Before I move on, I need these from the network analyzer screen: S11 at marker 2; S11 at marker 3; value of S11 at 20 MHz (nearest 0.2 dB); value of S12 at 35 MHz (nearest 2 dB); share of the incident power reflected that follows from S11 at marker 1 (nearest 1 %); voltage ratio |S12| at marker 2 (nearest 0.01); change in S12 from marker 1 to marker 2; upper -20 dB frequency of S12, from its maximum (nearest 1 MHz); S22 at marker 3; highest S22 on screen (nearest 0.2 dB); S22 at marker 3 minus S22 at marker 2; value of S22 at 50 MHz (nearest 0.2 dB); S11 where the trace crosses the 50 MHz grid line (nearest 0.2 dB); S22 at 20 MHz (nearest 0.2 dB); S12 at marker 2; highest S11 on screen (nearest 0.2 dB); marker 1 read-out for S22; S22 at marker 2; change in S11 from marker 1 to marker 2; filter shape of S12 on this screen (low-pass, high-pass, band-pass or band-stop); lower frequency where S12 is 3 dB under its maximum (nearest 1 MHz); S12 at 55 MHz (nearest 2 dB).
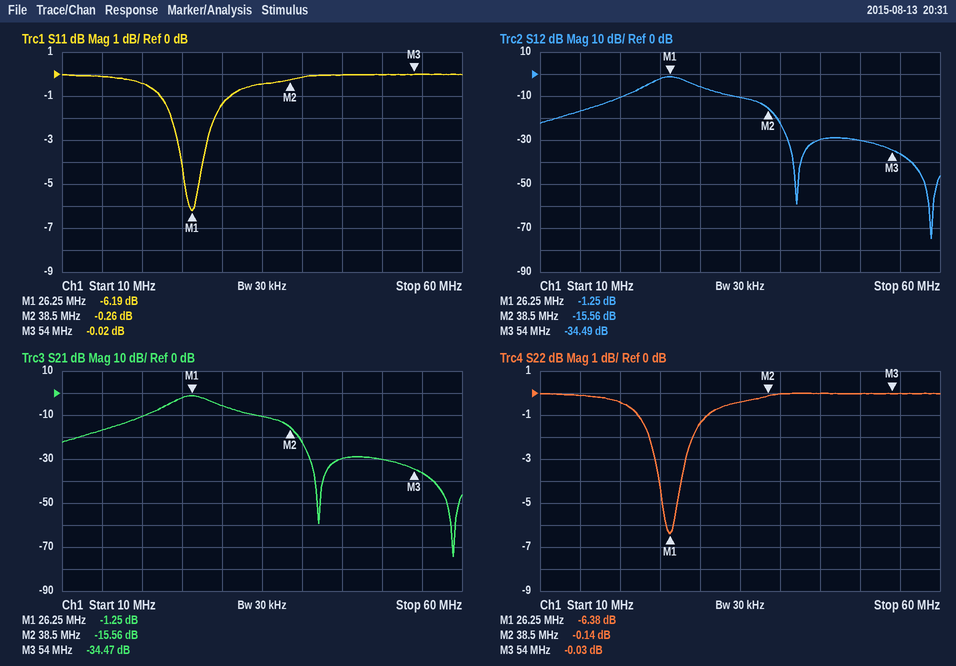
-0.26 dB
-0.02 dB
-0.4 dB
-10 dB
24 %
0.17
-14.31 dB
40 MHz
-0.03 dB
0.0 dB
0.11 dB
0.0 dB
0.0 dB
-0.4 dB
-15.56 dB
0.0 dB
-6.38 dB
-0.14 dB
5.93 dB
band-pass
24 MHz
-36 dB
